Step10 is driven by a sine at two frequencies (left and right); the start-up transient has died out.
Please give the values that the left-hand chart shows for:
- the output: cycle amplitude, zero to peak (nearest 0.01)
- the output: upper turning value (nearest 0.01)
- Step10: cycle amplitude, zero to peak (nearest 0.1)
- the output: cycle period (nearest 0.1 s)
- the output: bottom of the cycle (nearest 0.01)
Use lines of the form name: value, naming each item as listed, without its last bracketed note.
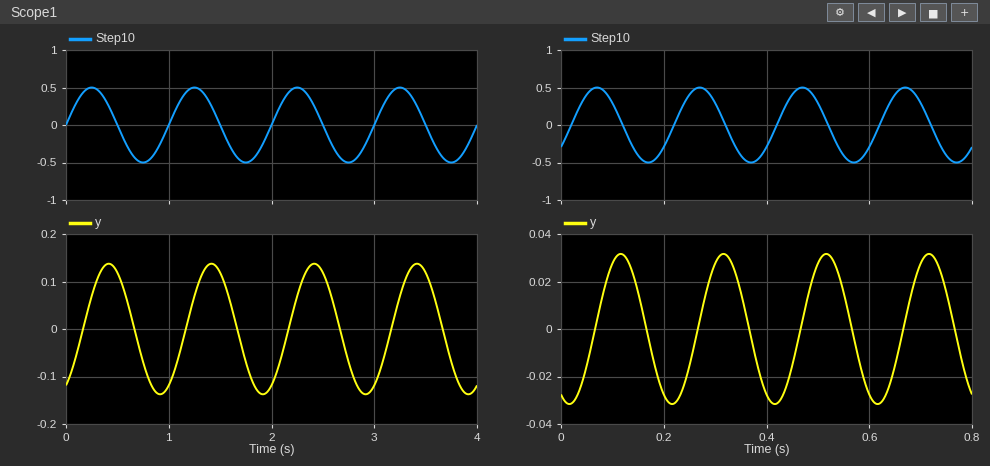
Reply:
the output: cycle amplitude, zero to peak: 0.14
the output: upper turning value: 0.14
Step10: cycle amplitude, zero to peak: 0.5
the output: cycle period: 1.0 s
the output: bottom of the cycle: -0.14
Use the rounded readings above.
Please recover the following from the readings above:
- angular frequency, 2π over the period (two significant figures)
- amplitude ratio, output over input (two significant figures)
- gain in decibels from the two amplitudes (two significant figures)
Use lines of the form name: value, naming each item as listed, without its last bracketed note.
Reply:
angular frequency, 2π over the period: 6.3 rad/s
amplitude ratio, output over input: 0.28
gain in decibels from the two amplitudes: -11 dB
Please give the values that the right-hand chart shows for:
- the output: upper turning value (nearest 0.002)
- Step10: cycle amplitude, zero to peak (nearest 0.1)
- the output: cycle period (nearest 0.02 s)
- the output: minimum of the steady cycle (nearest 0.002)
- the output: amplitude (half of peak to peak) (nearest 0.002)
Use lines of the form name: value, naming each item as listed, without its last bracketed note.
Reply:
the output: upper turning value: 0.032
Step10: cycle amplitude, zero to peak: 0.5
the output: cycle period: 0.20 s
the output: minimum of the steady cycle: -0.032
the output: amplitude (half of peak to peak): 0.032
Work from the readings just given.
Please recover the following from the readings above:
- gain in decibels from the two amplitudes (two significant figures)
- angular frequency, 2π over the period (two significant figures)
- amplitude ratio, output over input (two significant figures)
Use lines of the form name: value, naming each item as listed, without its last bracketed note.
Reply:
gain in decibels from the two amplitudes: -24 dB
angular frequency, 2π over the period: 31 rad/s
amplitude ratio, output over input: 0.064
